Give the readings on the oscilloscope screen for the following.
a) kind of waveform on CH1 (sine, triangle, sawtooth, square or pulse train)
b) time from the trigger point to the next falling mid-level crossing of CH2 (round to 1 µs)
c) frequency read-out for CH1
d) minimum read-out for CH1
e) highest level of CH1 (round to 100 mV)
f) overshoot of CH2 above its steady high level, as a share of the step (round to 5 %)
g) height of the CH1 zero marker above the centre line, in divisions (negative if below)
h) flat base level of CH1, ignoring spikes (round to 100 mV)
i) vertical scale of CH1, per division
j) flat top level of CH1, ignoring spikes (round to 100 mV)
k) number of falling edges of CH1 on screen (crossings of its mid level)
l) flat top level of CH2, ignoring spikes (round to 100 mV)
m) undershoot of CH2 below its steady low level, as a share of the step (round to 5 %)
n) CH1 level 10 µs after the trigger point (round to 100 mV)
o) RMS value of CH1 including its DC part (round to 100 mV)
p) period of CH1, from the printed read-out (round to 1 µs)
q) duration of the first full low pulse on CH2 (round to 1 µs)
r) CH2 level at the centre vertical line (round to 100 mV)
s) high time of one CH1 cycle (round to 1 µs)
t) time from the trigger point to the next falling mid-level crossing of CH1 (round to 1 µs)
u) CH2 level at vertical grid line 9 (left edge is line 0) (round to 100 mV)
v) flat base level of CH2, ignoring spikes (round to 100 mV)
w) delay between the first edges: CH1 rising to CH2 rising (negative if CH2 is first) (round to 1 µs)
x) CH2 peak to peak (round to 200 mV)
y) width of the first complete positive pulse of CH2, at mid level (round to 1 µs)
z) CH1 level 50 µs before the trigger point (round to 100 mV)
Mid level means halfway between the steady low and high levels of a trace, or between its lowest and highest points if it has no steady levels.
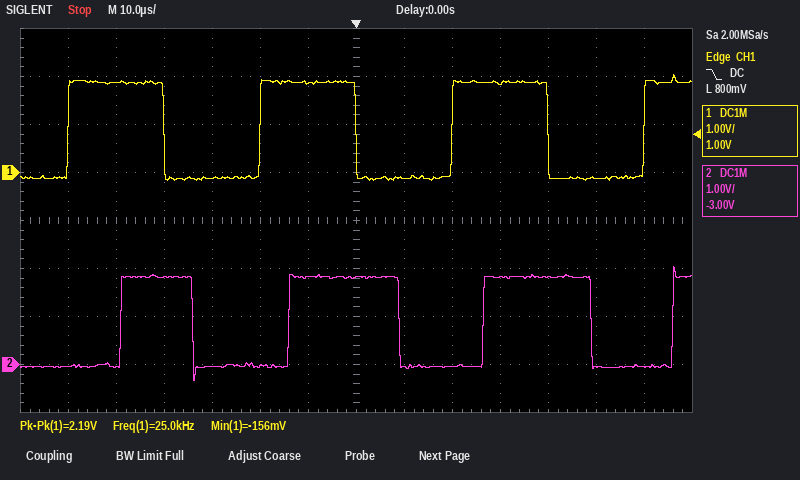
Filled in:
square
9 µs
25.0 kHz
-156 mV
2.0 V
10 %
+1.0 div
-100 mV
1 V
1.9 V
3
1.8 V
15 %
-100 mV
1.3 V
40 µs
20 µs
1.8 V
20 µs
40 µs
0.0 V
0.0 V
+11 µs
2.4 V
15 µs
1.9 V
